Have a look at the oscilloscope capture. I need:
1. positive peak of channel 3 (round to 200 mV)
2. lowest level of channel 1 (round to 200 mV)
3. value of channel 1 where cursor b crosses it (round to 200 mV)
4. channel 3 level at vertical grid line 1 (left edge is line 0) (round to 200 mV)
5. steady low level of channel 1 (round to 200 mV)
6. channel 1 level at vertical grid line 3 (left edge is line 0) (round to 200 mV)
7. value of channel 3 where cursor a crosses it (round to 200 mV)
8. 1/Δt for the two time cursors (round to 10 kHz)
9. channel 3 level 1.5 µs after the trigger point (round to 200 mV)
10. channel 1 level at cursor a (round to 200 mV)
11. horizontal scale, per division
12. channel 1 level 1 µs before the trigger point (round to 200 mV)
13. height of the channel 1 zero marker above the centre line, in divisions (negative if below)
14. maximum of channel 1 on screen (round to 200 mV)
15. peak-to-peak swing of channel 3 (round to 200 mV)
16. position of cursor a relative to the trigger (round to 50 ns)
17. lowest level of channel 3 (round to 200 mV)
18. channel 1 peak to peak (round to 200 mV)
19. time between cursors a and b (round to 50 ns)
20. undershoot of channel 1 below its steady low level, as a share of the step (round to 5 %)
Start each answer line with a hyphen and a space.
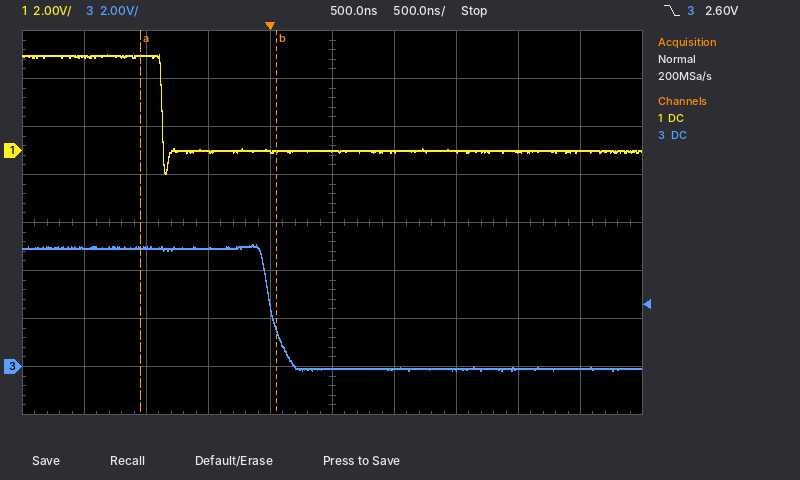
- 5.0 V
- -1.0 V
- 0.0 V
- 5.0 V
- 0.0 V
- 0.0 V
- 5.0 V
- 910 kHz
- -200 mV
- 4.0 V
- 500 ns
- 4.0 V
- +1.5 div
- 4.0 V
- 5.2 V
- -1.05 µs
- -200 mV
- 5.0 V
- 1.10 µs
- 25 %
